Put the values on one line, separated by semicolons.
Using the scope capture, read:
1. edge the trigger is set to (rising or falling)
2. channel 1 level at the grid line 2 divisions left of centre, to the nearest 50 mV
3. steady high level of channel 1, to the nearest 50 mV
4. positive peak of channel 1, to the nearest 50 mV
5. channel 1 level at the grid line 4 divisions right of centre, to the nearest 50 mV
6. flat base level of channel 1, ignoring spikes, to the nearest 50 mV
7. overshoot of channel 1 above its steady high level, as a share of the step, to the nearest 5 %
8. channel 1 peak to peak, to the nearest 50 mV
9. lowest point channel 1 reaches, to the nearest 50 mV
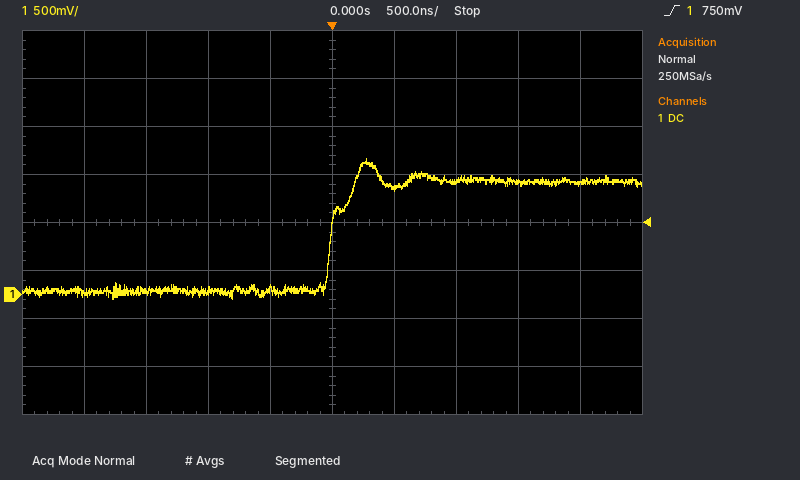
rising; 50 mV; 1.20 V; 1.40 V; 1.15 V; 50 mV; 20 %; 1.45 V; -50 mV
